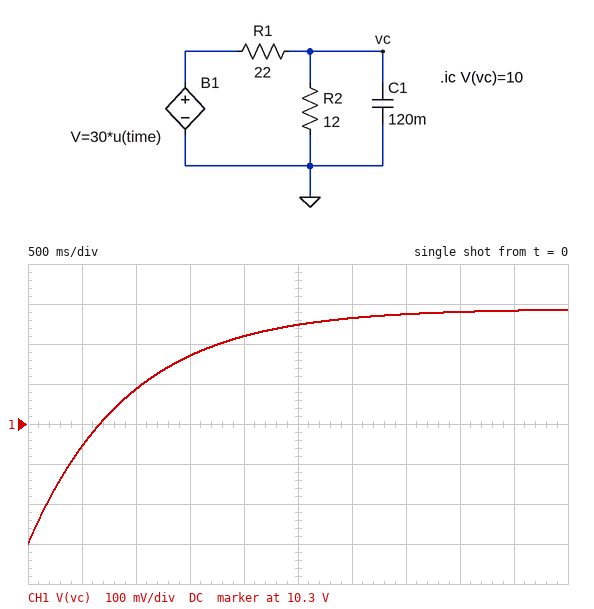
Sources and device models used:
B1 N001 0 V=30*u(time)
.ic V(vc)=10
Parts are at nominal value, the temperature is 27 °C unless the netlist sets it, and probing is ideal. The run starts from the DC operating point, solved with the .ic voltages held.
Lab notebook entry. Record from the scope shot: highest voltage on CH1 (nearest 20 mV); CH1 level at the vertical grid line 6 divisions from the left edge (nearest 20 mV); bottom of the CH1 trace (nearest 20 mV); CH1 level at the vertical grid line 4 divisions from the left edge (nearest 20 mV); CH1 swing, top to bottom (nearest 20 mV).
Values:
10.58 V
10.56 V
10.00 V
10.52 V
580 mV
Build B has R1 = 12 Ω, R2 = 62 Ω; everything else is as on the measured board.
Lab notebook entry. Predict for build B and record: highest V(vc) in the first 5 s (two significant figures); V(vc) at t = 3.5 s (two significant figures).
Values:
25 V
24 V
